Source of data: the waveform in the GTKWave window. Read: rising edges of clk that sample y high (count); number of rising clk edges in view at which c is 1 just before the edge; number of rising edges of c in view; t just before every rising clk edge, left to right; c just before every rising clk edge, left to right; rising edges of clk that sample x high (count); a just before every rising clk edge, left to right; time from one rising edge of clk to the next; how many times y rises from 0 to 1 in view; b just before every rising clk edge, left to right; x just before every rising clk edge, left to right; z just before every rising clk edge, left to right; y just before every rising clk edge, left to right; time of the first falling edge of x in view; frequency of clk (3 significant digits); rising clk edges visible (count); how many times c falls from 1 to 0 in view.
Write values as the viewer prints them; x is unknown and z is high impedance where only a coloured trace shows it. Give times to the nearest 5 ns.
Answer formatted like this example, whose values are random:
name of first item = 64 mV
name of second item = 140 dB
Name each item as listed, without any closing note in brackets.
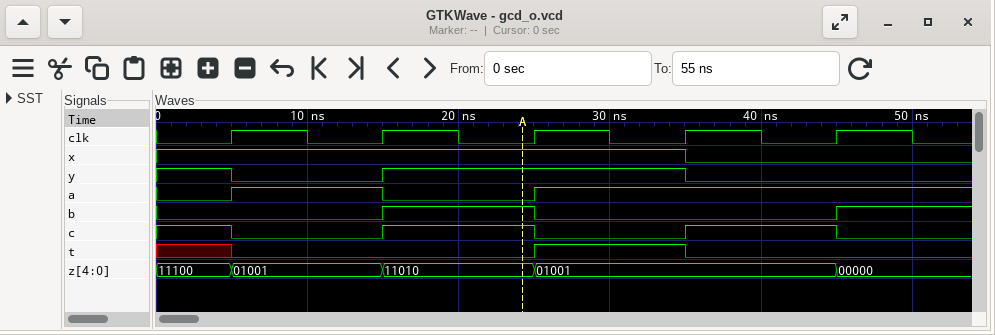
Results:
rising edges of clk that sample y high = 3
number of rising clk edges in view at which c is 1 just before the edge = 3
number of rising edges of c in view = 2
t just before every rising clk edge, left to right = x 0 0 1 0
c just before every rising clk edge, left to right = 1 0 1 0 1
rising edges of clk that sample x high = 4
a just before every rising clk edge, left to right = 0 1 0 1 1
time from one rising edge of clk to the next = 10 ns
how many times y rises from 0 to 1 in view = 1
b just before every rising clk edge, left to right = 0 0 1 0 0
x just before every rising clk edge, left to right = 1 1 1 1 0
z just before every rising clk edge, left to right = 11100, 01001, 11010, 01001, 01001
y just before every rising clk edge, left to right = 1 0 1 1 0
time of the first falling edge of x in view = 35 ns
frequency of clk = 100 MHz
rising clk edges visible = 5
how many times c falls from 1 to 0 in view = 3
